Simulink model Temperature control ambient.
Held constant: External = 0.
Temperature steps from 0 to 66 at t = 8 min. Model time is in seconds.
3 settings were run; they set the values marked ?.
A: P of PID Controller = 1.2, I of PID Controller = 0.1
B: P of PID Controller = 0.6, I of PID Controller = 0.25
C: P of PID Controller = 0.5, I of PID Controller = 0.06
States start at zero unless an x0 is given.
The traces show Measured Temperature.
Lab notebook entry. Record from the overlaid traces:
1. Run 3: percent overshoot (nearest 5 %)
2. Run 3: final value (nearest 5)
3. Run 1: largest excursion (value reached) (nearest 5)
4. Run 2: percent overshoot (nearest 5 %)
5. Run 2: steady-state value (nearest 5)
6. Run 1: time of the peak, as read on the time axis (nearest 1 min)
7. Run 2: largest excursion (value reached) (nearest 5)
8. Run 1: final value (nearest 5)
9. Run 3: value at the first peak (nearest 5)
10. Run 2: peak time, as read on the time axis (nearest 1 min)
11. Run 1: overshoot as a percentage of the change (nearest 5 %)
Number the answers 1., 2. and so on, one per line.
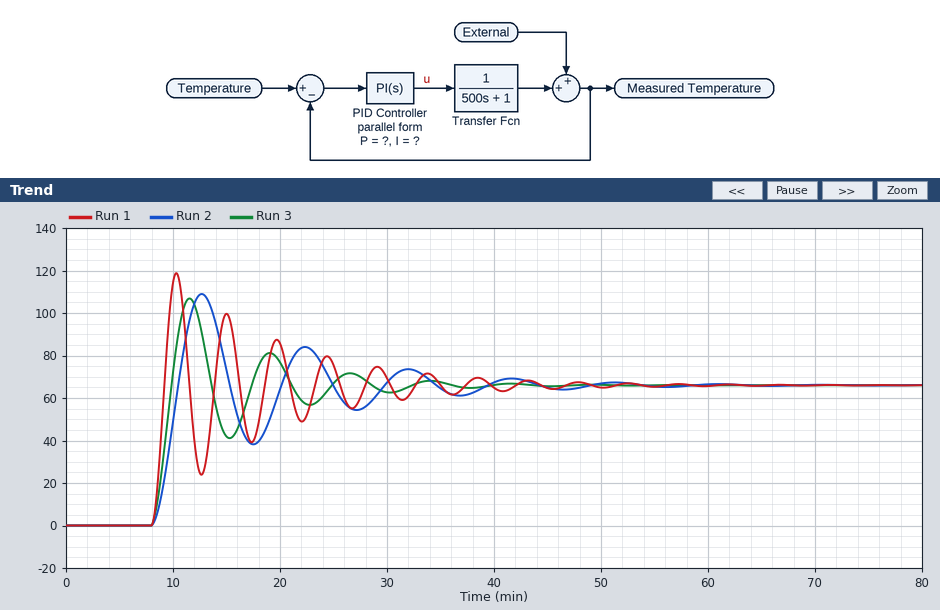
1. 60 %
2. 65
3. 120
4. 65 %
5. 65
6. 10 min
7. 110
8. 65
9. 105
10. 13 min
11. 80 %
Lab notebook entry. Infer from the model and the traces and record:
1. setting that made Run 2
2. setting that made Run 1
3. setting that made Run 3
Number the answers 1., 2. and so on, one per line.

1. C
2. B
3. A
